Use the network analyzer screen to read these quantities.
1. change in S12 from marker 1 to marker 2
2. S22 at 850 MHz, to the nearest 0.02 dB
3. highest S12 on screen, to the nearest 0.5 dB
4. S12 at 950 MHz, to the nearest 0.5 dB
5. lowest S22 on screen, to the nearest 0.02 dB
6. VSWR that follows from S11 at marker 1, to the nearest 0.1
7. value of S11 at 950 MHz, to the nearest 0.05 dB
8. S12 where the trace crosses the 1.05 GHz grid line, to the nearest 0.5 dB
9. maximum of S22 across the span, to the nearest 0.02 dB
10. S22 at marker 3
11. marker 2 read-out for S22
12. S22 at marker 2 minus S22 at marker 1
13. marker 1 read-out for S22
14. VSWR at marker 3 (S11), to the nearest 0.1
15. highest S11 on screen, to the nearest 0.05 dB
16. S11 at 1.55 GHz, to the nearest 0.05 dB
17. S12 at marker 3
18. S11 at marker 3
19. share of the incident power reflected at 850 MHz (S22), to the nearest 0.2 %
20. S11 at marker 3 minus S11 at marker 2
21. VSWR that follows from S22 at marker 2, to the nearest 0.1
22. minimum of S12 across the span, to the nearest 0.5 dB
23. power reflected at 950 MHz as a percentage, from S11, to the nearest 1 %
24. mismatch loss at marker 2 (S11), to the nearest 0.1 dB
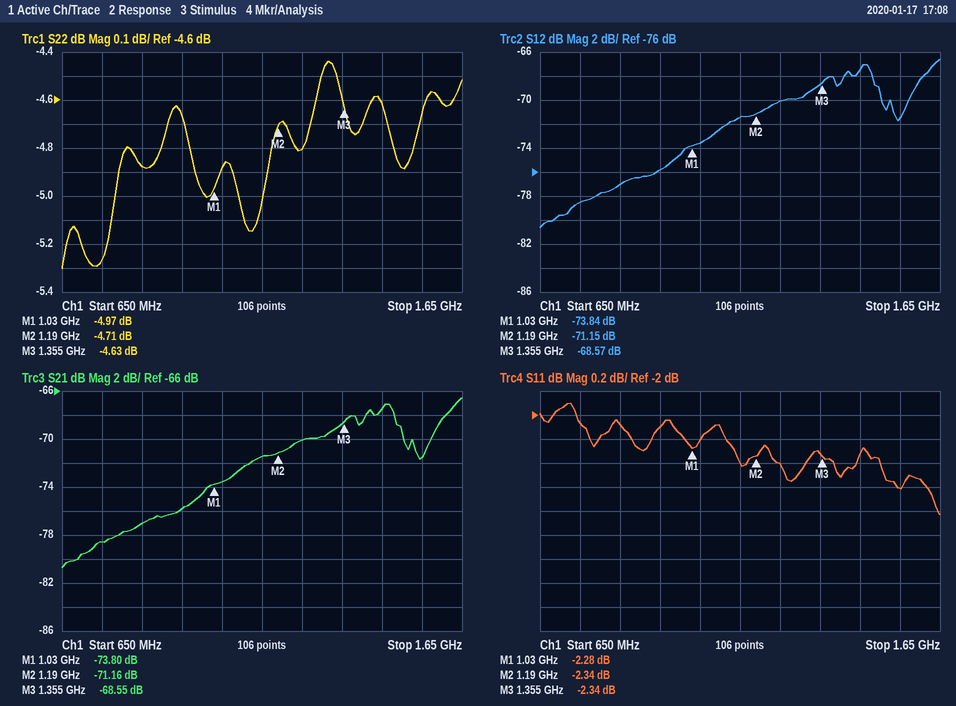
2.69 dB
-4.88 dB
-66.5 dB
-76.0 dB
-5.30 dB
7.7
-2.10 dB
-73.5 dB
-4.44 dB
-4.63 dB
-4.71 dB
0.26 dB
-4.97 dB
7.5
-1.90 dB
-2.60 dB
-68.57 dB
-2.34 dB
32.6 %
0.00 dB
3.8
-80.5 dB
62 %
3.8 dB
